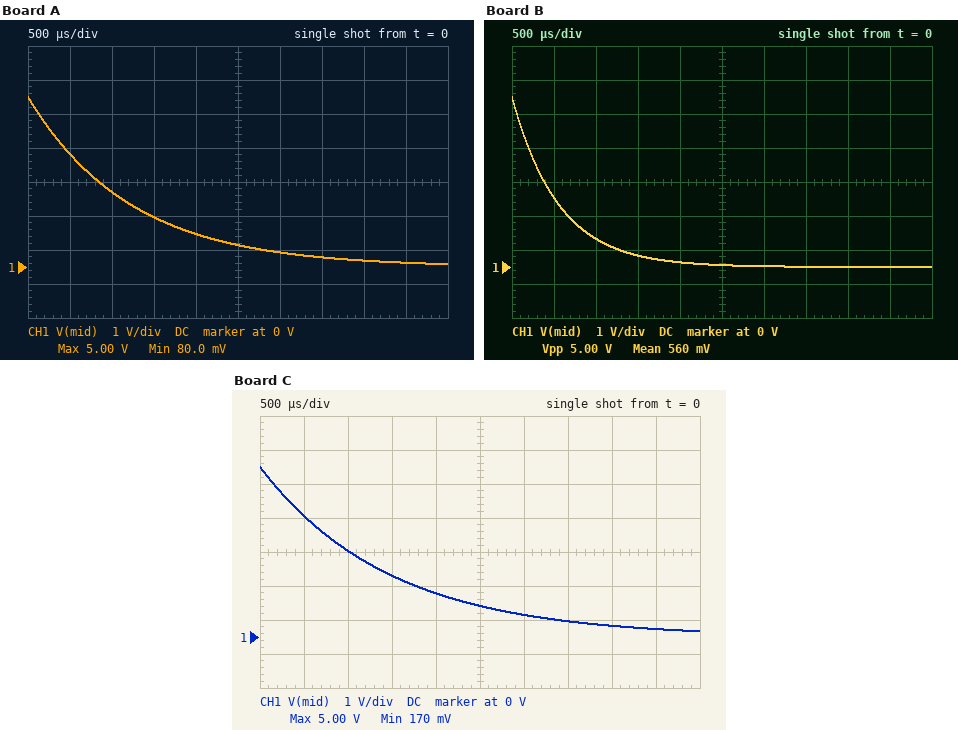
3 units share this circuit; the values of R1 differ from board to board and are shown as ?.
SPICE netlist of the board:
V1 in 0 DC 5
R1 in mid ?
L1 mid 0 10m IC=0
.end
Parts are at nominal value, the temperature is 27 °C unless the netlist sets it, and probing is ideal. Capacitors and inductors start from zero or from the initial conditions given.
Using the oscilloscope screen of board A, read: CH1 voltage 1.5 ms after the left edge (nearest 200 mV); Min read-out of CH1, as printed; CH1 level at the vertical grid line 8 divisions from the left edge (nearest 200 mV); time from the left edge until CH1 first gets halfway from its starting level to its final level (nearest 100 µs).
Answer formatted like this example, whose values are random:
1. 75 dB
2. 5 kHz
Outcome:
1. 1.4 V
2. 80.0 mV
3. 200 mV
4. 800 µs
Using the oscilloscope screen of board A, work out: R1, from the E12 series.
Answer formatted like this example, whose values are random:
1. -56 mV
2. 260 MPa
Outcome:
1. 8.2 Ω
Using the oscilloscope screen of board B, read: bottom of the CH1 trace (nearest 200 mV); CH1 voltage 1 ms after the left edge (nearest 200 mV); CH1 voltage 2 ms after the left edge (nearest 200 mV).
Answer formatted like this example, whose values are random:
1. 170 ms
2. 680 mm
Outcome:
1. 0 V
2. 800 mV
3. 200 mV
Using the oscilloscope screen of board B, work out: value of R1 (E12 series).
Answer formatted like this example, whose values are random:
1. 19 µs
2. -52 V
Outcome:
1. 18 Ω
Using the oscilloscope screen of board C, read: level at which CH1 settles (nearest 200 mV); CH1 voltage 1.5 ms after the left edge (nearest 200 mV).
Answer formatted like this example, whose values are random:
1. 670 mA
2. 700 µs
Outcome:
1. 200 mV
2. 1.8 V
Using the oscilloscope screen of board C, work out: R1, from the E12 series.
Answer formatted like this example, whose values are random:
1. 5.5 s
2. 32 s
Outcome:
1. 6.8 Ω
